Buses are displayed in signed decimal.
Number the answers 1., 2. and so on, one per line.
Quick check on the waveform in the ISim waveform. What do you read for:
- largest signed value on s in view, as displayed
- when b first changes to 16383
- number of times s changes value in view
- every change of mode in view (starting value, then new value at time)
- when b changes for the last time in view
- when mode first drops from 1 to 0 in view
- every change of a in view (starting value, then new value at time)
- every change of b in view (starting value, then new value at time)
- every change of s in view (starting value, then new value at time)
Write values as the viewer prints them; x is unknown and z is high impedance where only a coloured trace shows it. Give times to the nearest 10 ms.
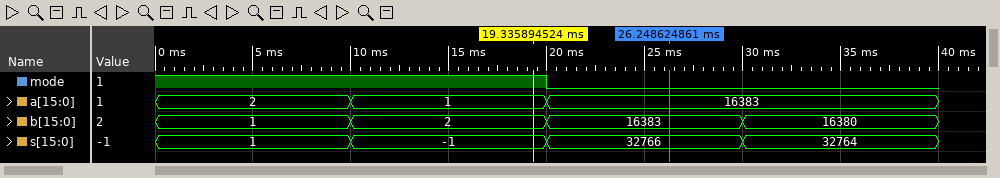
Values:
1. 32766
2. 20 ms
3. 3
4. 1, 0 at 20 ms
5. 30 ms
6. 20 ms
7. 2, 1 at 10 ms, 16383 at 20 ms
8. 1, 2 at 10 ms, 16383 at 20 ms, 16380 at 30 ms
9. 1, -1 at 10 ms, 32766 at 20 ms, 32764 at 30 ms
